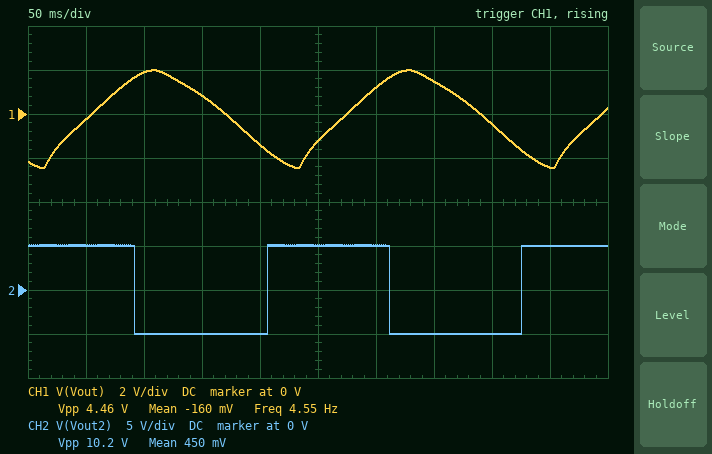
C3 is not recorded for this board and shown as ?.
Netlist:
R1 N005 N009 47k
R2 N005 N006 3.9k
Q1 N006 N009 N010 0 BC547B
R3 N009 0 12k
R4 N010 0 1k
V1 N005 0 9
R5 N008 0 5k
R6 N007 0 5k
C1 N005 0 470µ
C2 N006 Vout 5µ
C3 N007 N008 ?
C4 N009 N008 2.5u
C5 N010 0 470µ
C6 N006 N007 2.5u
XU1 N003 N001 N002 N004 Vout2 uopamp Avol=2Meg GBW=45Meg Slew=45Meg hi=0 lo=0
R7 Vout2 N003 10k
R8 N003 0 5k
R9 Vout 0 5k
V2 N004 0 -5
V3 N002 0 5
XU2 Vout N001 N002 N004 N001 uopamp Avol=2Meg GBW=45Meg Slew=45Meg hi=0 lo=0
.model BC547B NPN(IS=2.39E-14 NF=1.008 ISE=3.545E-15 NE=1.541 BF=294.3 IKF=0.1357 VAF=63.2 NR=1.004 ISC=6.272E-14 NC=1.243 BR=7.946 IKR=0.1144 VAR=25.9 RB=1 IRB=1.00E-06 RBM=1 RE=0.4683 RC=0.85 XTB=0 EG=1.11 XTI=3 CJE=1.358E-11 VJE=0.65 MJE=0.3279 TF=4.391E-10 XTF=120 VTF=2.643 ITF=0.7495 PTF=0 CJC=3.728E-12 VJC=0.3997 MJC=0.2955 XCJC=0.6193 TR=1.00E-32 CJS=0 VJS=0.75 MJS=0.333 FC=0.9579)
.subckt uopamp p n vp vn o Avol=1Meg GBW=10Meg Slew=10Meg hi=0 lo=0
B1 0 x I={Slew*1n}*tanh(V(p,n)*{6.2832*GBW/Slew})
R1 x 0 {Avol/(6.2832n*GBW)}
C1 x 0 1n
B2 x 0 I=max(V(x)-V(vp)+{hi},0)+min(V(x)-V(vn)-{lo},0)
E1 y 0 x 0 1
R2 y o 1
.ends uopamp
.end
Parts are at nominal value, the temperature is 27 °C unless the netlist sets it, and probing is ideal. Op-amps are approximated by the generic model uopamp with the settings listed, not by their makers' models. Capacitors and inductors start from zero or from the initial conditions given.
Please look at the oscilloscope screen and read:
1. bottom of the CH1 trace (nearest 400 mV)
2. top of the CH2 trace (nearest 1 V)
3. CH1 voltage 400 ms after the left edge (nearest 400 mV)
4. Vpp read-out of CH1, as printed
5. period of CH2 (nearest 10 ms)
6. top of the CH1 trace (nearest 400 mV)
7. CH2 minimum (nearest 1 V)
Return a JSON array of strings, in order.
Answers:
["-2.4 V", "5 V", "-400 mV", "4.46 V", "220 ms", "2.0 V", "-5 V"]
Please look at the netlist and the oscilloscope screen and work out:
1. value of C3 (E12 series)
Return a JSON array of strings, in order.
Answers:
["4.7 µF"]
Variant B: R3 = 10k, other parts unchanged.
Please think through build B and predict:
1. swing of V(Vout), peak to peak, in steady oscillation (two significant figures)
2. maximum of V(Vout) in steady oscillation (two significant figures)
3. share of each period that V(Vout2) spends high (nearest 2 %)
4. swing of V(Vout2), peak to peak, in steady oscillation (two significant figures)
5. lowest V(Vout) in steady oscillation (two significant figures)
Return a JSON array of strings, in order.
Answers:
["3.8 V", "2.1 V", "36 %", "10 V", "-1.7 V"]
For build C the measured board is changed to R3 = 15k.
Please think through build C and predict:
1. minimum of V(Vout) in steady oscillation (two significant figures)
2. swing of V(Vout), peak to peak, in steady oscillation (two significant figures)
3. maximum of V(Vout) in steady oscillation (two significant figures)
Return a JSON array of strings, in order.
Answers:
["-1.6 V", "2.6 V", "1.0 V"]
